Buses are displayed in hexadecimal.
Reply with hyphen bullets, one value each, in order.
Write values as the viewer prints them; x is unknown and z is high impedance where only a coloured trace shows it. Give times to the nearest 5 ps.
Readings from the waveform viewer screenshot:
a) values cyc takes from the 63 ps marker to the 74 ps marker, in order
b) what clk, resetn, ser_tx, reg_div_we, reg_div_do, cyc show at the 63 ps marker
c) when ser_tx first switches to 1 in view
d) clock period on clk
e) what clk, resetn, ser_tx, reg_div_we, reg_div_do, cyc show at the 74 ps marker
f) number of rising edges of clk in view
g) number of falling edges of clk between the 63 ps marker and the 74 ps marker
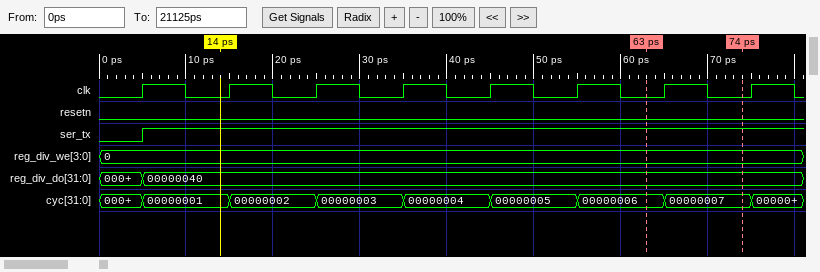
- 00000006, 00000007
- clk=0, resetn=0, ser_tx=1, reg_div_we=0, reg_div_do=00000040, cyc=00000006
- 5 ps
- 10 ps
- clk=0, resetn=0, ser_tx=1, reg_div_we=0, reg_div_do=00000040, cyc=00000007
- 8
- 1
